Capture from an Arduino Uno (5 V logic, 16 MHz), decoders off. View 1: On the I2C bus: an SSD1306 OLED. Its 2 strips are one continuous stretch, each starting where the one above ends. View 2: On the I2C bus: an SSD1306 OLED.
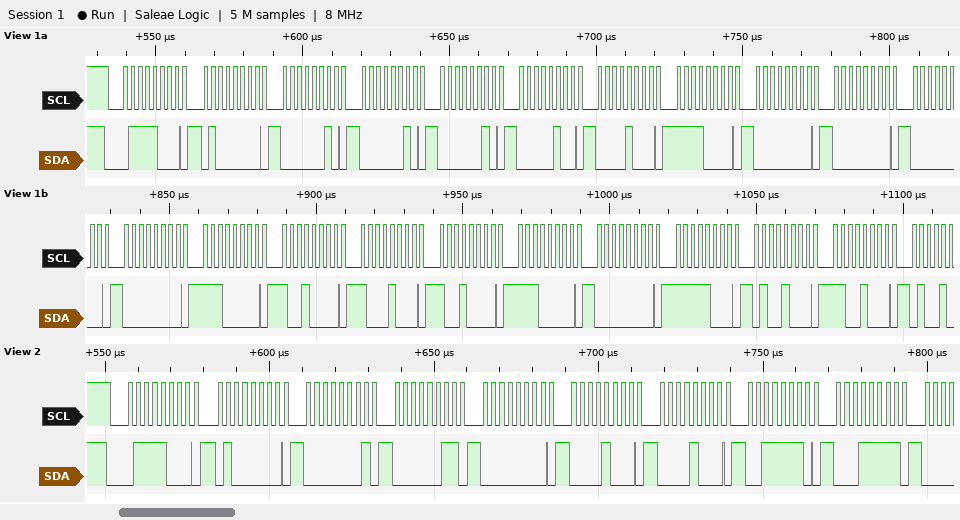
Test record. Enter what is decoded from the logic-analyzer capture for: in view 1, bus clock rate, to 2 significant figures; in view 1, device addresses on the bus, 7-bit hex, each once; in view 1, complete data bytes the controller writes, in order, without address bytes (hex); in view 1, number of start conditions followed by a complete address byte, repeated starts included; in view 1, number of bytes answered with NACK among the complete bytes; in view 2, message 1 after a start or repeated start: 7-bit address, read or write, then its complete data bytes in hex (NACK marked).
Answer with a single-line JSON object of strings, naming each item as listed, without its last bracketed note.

{"in view 1, bus clock rate, to 2 significant figures": "400 kHz", "in view 1, device addresses on the bus, 7-bit hex, each once": "0x3C", "in view 1, complete data bytes the controller writes, in order, without address bytes": "40 02 02 02 04 08 F0 00 00 00 00 E0 90 88 90 E0 00 F8 48 C8", "in view 1, number of start conditions followed by a complete address byte, repeated starts included": "1", "in view 1, number of bytes answered with NACK among the complete bytes": "0", "in view 2, message 1 after a start or repeated start: 7-bit address, read or write, then its complete data bytes in hex": "0x3C write: 40 01 03 00 08 08 3E 1F"}
